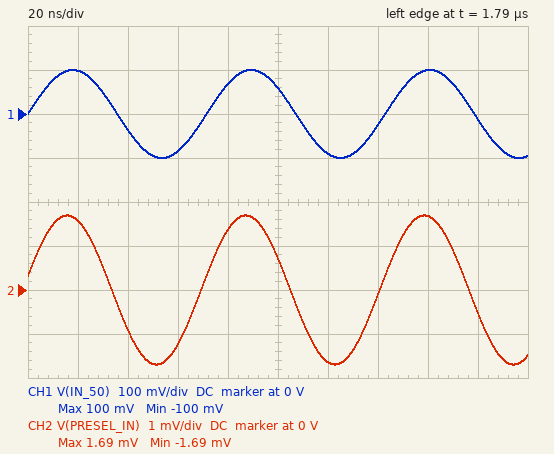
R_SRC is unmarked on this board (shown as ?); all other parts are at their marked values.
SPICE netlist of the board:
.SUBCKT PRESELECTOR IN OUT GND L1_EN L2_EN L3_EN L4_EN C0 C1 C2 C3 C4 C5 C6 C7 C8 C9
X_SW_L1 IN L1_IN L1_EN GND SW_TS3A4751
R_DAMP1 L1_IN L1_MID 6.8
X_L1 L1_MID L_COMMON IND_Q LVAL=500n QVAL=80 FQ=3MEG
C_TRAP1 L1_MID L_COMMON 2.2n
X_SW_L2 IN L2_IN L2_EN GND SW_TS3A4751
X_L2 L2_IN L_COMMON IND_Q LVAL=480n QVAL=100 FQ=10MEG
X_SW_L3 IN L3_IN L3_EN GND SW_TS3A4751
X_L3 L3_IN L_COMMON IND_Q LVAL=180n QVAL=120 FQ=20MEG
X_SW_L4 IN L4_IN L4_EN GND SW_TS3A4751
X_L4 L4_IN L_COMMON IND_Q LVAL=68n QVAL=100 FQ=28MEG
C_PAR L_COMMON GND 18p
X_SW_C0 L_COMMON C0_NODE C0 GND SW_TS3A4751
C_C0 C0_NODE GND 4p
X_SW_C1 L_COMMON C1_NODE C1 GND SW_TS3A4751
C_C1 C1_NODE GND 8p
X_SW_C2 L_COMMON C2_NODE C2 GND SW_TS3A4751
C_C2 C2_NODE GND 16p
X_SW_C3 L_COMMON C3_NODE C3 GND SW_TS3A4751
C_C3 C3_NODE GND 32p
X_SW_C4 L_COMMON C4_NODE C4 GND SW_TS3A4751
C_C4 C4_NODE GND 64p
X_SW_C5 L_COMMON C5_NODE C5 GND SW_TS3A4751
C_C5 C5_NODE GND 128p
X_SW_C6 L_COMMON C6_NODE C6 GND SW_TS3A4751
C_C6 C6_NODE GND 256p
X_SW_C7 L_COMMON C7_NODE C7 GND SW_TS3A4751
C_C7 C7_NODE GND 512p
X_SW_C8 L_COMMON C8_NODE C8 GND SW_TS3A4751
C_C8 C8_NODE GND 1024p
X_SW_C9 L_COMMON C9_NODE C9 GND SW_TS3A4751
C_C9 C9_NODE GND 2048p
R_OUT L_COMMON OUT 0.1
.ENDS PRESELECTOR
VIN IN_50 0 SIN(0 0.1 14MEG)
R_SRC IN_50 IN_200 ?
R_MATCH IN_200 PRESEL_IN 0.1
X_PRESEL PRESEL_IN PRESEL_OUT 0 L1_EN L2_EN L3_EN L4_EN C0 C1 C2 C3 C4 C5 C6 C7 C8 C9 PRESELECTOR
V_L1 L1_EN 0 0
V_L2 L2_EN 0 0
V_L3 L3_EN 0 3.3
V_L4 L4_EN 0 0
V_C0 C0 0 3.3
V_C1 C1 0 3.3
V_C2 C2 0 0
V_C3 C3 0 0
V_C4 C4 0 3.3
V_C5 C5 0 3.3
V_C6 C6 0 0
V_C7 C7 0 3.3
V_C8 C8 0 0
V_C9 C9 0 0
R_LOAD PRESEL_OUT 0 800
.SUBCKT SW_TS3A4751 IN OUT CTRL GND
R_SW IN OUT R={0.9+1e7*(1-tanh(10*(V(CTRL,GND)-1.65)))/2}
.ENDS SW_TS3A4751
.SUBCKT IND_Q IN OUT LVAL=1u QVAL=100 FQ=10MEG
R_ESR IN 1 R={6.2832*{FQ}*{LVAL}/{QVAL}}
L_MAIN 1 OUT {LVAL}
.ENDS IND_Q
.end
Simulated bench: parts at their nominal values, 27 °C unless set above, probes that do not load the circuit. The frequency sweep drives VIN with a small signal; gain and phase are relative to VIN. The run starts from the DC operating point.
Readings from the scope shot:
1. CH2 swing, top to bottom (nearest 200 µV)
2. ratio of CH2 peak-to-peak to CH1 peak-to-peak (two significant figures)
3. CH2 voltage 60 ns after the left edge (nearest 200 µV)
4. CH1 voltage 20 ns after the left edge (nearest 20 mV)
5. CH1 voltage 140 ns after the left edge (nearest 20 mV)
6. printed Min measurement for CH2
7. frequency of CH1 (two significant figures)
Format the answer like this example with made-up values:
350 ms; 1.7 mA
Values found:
3.4 mV; 0.017; -1.2 mV; 100 mV; -20 mV; -1.69 mV; 14 MHz
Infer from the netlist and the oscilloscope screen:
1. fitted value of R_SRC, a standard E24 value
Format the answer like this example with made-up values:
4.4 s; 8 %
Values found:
110 Ω
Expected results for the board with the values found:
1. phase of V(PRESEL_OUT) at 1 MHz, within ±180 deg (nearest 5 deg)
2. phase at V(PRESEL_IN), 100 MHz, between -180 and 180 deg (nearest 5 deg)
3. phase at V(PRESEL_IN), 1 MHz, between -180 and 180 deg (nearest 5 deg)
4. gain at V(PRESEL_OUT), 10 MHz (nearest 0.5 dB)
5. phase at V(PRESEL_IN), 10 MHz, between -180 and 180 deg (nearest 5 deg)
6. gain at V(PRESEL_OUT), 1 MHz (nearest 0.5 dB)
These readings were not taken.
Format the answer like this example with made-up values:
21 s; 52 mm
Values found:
-25 deg; 45 deg; -25 deg; -14.5 dB; -75 deg; -2.0 dB
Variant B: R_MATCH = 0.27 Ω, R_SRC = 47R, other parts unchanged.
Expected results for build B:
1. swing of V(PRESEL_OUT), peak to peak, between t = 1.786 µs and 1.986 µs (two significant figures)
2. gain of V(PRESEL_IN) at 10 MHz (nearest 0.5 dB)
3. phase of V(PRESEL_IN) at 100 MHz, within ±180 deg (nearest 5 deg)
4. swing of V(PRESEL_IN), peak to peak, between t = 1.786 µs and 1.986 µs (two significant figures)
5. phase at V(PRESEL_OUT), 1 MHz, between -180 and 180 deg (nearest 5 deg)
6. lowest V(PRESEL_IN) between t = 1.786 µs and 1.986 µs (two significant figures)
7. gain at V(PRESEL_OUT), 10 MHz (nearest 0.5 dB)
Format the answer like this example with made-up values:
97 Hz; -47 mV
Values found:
63 mV; -13.5 dB; 25 deg; 7.7 mV; -10 deg; -3.9 mV; -7.5 dB
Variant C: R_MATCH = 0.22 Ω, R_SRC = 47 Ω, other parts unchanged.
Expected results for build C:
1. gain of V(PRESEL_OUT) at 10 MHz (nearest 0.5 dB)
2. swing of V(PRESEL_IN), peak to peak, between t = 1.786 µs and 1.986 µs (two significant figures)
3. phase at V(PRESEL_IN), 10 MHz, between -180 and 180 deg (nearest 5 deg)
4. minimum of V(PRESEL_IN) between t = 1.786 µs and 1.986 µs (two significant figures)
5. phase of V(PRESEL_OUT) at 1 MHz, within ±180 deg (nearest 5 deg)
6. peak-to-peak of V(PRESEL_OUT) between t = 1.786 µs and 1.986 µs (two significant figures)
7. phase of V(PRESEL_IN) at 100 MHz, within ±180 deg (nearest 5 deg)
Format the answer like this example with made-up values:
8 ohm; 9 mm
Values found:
-7.5 dB; 7.7 mV; -65 deg; -3.9 mV; -10 deg; 63 mV; 25 deg
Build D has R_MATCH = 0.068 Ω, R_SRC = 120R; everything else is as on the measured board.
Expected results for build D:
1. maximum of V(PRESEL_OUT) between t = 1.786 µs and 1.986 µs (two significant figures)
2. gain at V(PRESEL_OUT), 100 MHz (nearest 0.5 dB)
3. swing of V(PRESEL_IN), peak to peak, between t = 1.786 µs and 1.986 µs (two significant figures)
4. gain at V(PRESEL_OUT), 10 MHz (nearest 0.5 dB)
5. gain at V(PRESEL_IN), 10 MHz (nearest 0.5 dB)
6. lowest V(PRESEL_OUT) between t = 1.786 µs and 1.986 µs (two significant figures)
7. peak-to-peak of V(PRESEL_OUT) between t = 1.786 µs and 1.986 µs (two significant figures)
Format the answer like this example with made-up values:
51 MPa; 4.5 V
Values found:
13 mV; -37.5 dB; 3.1 mV; -15.0 dB; -21.5 dB; -13 mV; 25 mV
